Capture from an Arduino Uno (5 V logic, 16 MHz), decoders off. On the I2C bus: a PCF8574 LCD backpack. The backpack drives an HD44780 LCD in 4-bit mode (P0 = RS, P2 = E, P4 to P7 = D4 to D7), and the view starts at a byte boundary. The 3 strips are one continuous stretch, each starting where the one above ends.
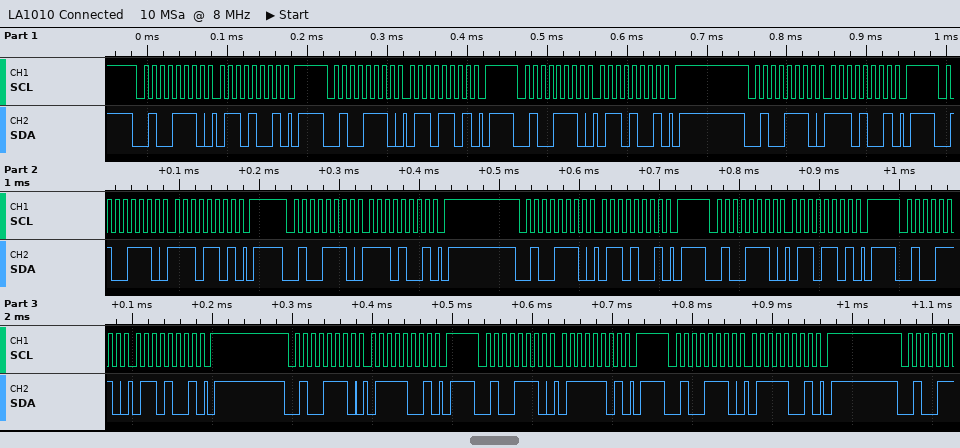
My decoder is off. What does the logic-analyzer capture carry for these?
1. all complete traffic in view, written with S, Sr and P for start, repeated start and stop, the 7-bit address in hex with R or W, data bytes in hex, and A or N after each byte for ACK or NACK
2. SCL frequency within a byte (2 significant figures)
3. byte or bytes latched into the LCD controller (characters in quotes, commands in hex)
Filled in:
S 27W A 69 A P S 27W A 6D A P S 27W A 69 A P S 27W A E9 A P S 27W A ED A P S 27W A E9 A P S 27W A 69 A P S 27W A 6D A P S 27W A 69 A P S 27W A 79 A P S 27W A 7D A P S 27W A 79 A P
100 kHz
'n' 'g'
